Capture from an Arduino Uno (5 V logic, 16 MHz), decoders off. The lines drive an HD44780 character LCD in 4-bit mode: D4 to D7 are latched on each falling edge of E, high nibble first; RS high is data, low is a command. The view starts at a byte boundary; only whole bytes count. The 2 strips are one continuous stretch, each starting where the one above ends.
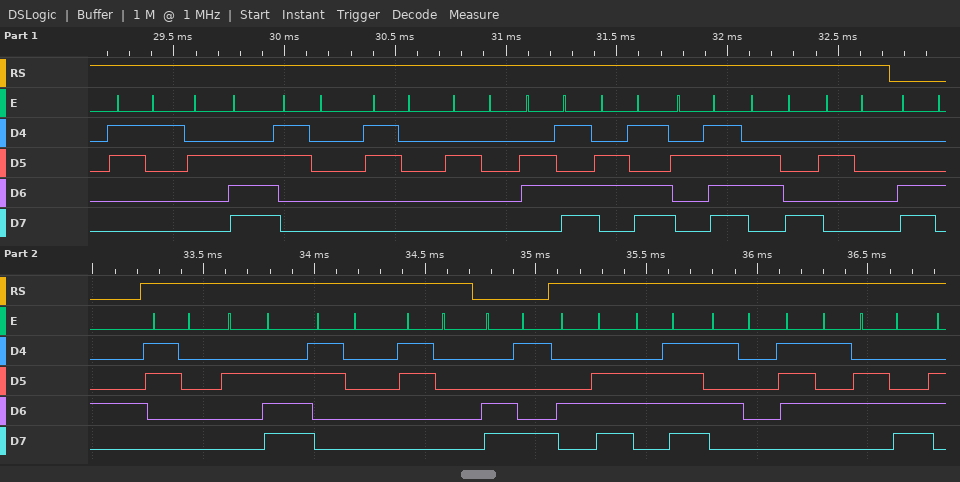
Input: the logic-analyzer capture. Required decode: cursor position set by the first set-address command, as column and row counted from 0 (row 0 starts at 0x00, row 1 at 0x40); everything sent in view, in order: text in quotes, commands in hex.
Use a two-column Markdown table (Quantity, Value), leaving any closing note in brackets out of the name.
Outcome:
| Quantity | Value |
|---|---|
| cursor position set by the first set-address command, as column and row counted from 0 | column 4, row 1 |
| everything sent in view, in order: text in quotes, commands in hex | "1.00 mm/h " 0xC4 "0.00" 0xC9 "NoPul" |
